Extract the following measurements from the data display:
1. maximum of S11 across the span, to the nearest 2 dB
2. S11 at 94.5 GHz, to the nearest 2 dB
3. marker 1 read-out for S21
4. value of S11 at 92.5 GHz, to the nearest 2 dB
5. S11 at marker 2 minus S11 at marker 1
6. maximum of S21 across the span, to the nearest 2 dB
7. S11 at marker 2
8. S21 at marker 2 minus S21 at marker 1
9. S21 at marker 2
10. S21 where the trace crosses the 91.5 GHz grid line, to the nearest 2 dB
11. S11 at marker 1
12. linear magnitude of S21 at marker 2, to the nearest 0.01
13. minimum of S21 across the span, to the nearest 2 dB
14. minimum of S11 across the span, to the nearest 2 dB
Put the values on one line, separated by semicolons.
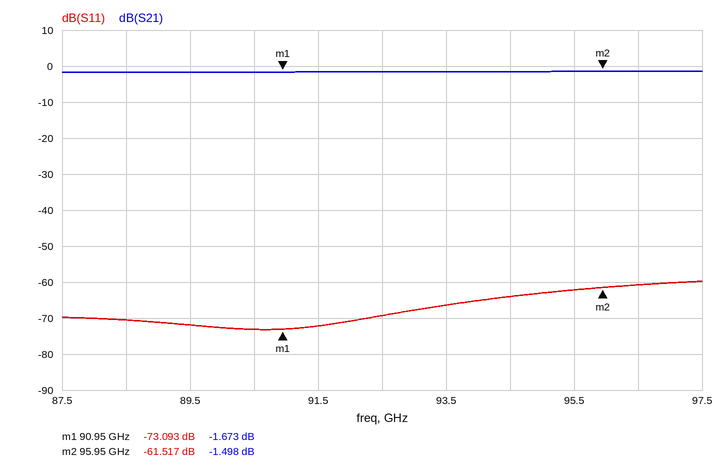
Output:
-60 dB; -64 dB; -1.673 dB; -70 dB; 11.576 dB; -2 dB; -61.517 dB; 0.175 dB; -1.498 dB; -2 dB; -73.093 dB; 0.84; -2 dB; -74 dB
